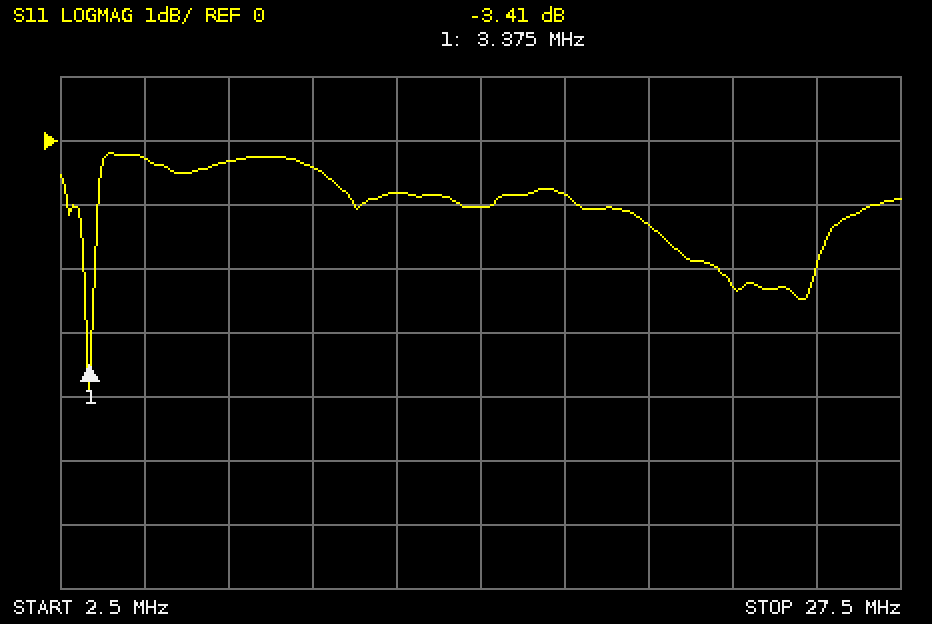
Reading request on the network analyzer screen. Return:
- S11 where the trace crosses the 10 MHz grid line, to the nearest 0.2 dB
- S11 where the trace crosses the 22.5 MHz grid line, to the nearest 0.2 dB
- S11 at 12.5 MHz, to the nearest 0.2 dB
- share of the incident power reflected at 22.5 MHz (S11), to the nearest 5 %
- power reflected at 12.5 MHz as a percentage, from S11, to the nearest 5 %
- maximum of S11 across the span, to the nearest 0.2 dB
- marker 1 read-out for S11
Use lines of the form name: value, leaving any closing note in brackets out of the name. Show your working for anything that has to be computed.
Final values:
S11 where the trace crosses the 10 MHz grid line, to the nearest 0.2 dB: -0.4 dB
S11 where the trace crosses the 22.5 MHz grid line, to the nearest 0.2 dB: -2.2 dB
S11 at 12.5 MHz, to the nearest 0.2 dB: -0.8 dB
share of the incident power reflected at 22.5 MHz (S11), to the nearest 5 %: 10^(-2.2/10) ≈ 60 %
power reflected at 12.5 MHz as a percentage, from S11, to the nearest 5 %: 10^(-0.8/10) ≈ 83.2 %, so 85 % to the nearest 5 %
maximum of S11 across the span, to the nearest 0.2 dB: -0.2 dB
marker 1 read-out for S11: -3.41 dB
